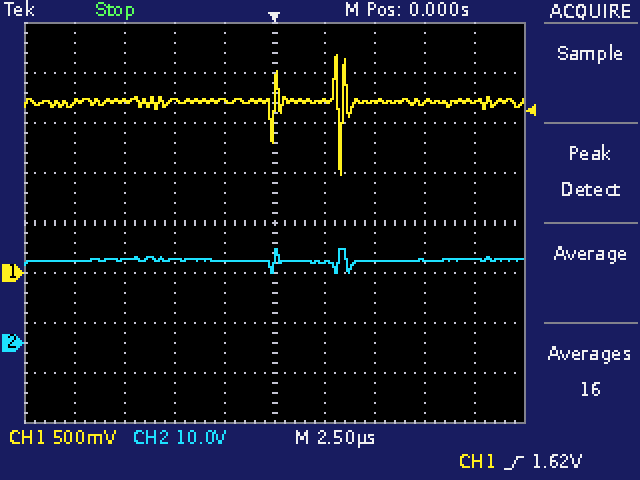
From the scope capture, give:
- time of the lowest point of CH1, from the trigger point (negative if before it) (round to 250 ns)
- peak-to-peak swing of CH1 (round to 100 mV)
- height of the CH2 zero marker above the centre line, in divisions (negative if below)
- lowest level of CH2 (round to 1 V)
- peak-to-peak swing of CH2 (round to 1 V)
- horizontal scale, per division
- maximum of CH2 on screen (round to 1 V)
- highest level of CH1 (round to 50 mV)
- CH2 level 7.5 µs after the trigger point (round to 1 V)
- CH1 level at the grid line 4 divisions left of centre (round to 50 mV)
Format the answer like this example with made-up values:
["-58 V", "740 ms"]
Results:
["+3.25 µs", "1.20 V", "-2.4 div", "14 V", "5 V", "2.5 µs", "19 V", "2.20 V", "17 V", "1.70 V"]
